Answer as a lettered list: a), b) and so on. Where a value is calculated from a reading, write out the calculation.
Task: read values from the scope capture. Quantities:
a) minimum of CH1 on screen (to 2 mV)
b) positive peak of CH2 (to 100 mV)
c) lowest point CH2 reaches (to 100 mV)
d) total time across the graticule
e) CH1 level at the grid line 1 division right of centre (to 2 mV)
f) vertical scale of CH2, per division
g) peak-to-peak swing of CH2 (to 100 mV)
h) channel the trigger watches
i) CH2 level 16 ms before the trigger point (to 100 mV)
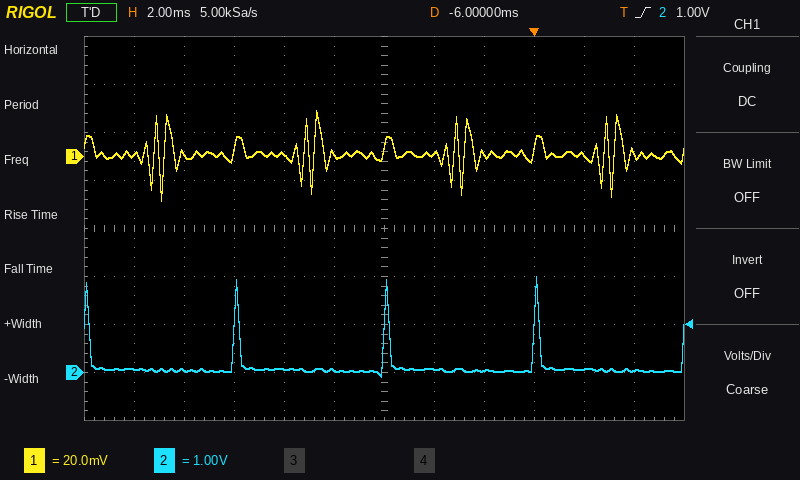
a) -18 mV
b) 2.0 V
c) -100 mV
d) 24 ms
e) 2 mV
f) 1 V
g) 2.0 V − (-100 mV) = 2.1 V
h) CH2
i) 100 mV
